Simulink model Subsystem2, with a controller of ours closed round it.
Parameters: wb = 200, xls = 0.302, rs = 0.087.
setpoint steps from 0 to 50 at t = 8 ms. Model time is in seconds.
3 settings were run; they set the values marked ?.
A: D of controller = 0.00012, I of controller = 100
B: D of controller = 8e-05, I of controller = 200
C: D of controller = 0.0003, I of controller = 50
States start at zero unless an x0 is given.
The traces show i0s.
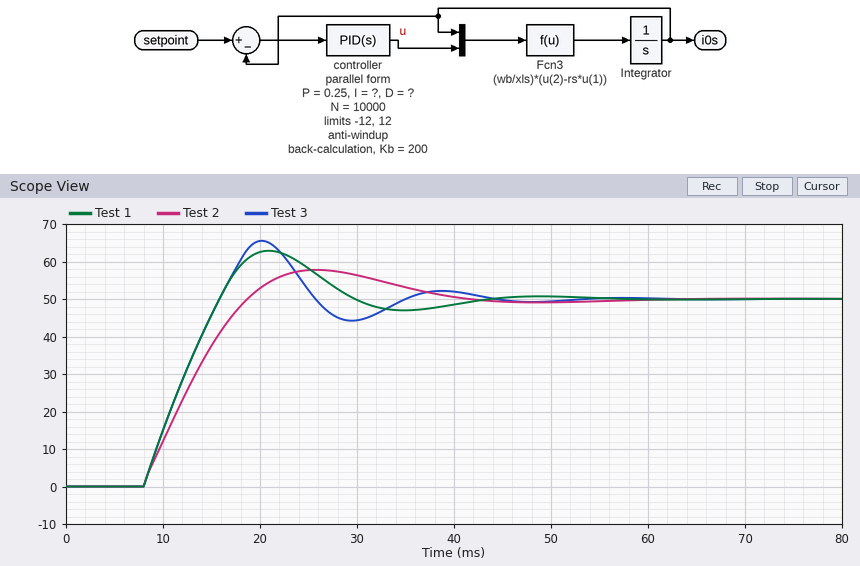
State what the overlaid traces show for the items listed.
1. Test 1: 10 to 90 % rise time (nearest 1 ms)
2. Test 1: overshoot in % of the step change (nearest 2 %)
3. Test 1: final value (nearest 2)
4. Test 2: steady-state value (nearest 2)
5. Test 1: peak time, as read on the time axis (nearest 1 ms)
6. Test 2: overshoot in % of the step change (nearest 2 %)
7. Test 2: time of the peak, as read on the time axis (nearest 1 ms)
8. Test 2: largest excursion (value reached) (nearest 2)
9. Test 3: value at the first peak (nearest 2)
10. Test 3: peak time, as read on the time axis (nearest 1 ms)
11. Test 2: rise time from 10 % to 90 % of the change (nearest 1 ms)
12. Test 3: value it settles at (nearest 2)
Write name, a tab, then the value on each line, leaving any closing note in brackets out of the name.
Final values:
Test 1: 10 to 90 % rise time	6 ms
Test 1: overshoot in % of the step change	26 %
Test 1: final value	50
Test 2: steady-state value	50
Test 1: peak time, as read on the time axis	21 ms
Test 2: overshoot in % of the step change	16 %
Test 2: time of the peak, as read on the time axis	26 ms
Test 2: largest excursion (value reached)	58
Test 3: value at the first peak	66
Test 3: peak time, as read on the time axis	20 ms
Test 2: rise time from 10 % to 90 % of the change	8 ms
Test 3: value it settles at	50
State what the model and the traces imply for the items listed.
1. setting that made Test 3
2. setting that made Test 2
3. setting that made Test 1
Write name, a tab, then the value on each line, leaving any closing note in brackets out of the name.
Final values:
setting that made Test 3	B
setting that made Test 2	C
setting that made Test 1	A
